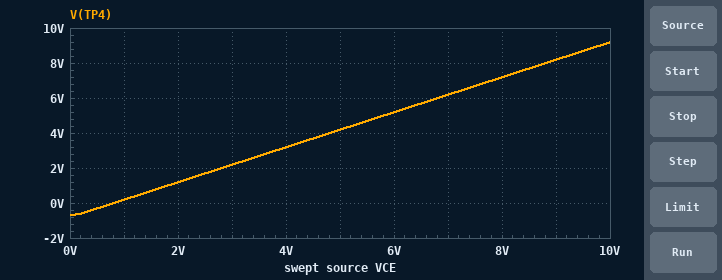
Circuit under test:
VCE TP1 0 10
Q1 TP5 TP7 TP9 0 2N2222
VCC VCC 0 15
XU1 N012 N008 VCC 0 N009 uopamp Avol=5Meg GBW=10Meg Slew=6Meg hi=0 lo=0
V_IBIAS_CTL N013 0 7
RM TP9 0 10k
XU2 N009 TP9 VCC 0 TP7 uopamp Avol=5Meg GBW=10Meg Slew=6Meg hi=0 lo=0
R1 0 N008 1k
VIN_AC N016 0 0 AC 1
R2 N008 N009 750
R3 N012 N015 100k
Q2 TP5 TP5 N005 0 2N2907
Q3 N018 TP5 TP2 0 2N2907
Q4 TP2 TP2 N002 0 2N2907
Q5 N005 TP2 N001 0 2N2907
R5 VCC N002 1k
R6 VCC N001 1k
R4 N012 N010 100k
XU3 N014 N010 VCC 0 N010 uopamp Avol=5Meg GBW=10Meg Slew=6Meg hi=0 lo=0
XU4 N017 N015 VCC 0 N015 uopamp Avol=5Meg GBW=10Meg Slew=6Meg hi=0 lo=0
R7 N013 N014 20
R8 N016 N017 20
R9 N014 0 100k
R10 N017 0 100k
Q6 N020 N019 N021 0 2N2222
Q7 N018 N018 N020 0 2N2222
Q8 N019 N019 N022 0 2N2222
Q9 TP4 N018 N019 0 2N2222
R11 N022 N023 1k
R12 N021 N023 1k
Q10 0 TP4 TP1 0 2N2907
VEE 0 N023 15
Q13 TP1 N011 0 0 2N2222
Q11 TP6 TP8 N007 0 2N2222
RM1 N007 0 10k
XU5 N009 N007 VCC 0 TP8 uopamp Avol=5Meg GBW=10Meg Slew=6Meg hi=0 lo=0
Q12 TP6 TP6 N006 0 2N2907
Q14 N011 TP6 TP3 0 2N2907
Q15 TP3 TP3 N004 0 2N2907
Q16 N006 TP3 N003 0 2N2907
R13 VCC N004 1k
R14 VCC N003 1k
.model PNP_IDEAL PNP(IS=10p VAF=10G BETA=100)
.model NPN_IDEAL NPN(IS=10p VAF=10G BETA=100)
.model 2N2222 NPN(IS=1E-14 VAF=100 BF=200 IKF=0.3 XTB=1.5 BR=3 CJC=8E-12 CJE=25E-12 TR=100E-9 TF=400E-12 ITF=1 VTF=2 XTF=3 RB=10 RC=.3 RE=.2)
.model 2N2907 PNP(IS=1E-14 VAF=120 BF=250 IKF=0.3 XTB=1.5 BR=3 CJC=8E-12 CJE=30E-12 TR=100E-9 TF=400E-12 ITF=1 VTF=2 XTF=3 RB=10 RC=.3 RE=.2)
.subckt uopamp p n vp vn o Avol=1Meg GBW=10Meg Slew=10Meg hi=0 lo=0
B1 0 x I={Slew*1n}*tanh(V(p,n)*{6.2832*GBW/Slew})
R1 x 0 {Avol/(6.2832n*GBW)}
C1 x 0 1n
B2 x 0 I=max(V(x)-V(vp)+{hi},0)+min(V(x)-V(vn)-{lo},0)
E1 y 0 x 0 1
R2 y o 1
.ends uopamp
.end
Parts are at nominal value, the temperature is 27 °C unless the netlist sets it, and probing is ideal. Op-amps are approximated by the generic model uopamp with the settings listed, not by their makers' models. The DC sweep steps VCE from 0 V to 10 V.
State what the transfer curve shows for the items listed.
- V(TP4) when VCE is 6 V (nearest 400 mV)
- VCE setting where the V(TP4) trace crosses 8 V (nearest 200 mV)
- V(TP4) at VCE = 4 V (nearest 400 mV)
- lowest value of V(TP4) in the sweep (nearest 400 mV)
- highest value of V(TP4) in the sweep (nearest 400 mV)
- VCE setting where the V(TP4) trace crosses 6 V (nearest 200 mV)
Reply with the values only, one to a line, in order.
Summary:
5.2 V
8.8 V
3.2 V
-800 mV
9.2 V
6.8 V
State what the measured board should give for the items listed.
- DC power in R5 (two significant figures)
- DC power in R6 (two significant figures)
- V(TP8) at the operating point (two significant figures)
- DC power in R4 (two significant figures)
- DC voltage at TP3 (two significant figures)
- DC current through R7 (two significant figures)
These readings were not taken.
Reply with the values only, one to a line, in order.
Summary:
370 µW
370 µW
6.8 V
120 µW
14 V
70 µA
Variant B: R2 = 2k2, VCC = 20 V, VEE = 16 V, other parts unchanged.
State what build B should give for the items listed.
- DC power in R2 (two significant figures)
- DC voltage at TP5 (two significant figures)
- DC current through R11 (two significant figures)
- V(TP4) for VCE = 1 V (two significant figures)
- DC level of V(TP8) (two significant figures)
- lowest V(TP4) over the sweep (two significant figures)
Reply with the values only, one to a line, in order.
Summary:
27 mW
18 V
1.1 mA
150 mV
12 V
-700 mV
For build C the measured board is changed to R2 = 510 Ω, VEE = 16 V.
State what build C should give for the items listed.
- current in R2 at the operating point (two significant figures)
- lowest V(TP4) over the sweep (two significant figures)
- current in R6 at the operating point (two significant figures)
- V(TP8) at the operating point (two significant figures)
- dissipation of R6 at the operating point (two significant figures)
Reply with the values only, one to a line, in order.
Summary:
3.5 mA
-670 mV
530 µA
5.9 V
280 µW
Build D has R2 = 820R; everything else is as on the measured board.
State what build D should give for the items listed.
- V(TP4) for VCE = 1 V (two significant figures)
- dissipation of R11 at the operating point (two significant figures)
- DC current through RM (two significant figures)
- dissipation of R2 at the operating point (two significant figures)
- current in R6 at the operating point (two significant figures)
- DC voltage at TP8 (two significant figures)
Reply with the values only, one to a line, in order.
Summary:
180 mV
400 µW
640 µA
10 mW
630 µA
7.0 V
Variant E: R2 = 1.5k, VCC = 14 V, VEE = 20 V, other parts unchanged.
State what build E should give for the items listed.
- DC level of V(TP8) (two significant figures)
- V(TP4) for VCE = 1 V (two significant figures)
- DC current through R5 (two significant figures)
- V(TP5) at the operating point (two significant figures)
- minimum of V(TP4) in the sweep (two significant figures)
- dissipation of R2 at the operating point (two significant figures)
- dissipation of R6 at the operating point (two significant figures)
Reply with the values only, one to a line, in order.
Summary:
9.4 V
170 mV
870 µA
12 V
-690 mV
18 mW
760 µW
